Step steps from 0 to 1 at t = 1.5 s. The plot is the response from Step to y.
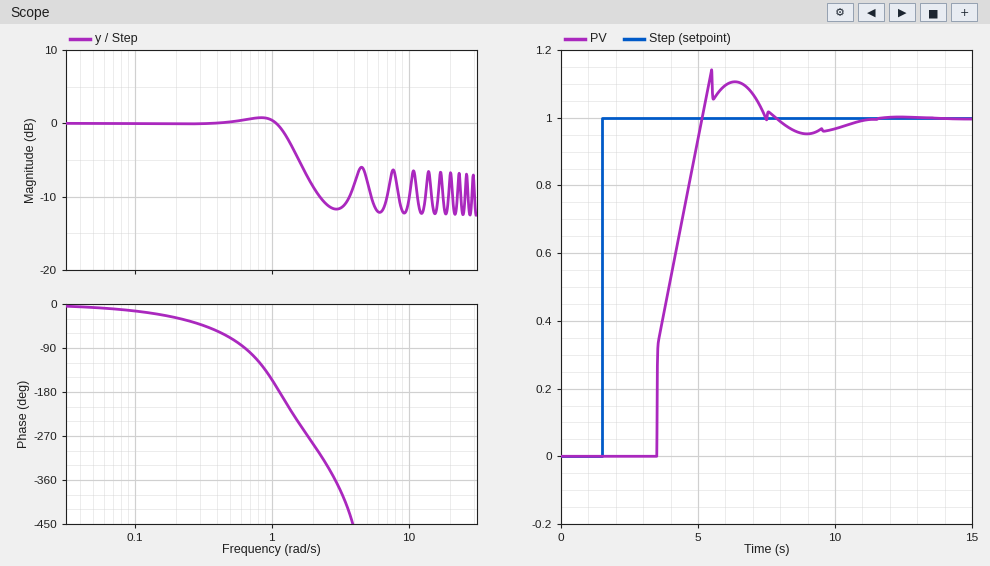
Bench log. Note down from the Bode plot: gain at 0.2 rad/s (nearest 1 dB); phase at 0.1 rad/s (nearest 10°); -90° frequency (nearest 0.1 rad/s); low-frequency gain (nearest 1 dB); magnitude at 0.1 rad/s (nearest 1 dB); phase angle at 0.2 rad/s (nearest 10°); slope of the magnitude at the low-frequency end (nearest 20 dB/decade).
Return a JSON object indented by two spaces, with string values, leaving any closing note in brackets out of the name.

{
  "gain at 0.2 rad/s": "0 dB",
  "phase at 0.1 rad/s": "-10°",
  "-90° frequency": "0.6 rad/s",
  "low-frequency gain": "0 dB",
  "magnitude at 0.1 rad/s": "0 dB",
  "phase angle at 0.2 rad/s": "-30°",
  "slope of the magnitude at the low-frequency end": "0 dB/decade"
}
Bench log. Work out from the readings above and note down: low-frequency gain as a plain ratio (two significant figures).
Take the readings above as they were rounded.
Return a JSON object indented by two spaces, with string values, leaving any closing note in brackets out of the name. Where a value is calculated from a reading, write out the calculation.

{
  "low-frequency gain as a plain ratio": "10^(0 / 20) = 1.0"
}
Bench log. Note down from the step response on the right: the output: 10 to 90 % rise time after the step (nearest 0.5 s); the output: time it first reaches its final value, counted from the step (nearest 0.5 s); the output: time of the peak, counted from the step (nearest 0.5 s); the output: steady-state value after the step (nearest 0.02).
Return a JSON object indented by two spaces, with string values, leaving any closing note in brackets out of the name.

{
  "the output: 10 to 90 % rise time after the step": "1.5 s",
  "the output: time it first reaches its final value, counted from the step": "3.5 s",
  "the output: time of the peak, counted from the step": "4.0 s",
  "the output: steady-state value after the step": "1.00"
}
